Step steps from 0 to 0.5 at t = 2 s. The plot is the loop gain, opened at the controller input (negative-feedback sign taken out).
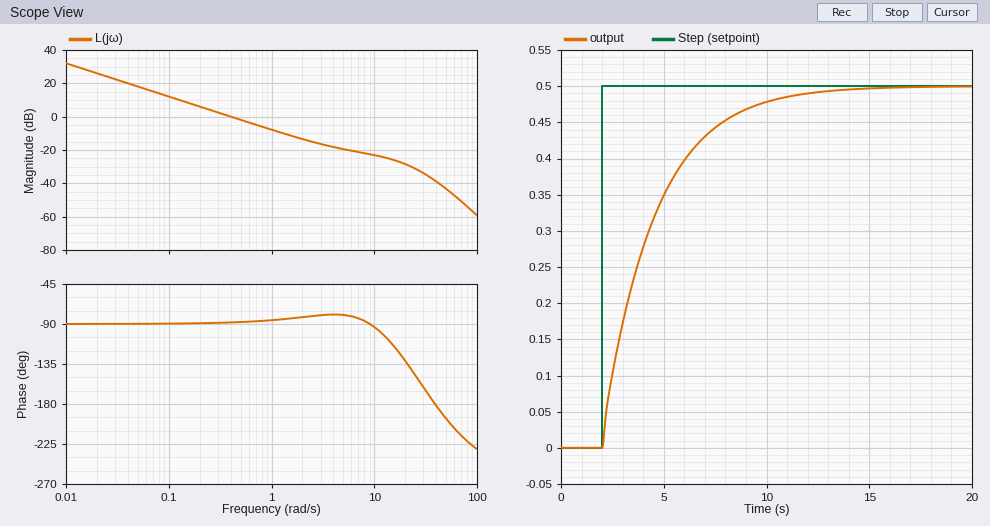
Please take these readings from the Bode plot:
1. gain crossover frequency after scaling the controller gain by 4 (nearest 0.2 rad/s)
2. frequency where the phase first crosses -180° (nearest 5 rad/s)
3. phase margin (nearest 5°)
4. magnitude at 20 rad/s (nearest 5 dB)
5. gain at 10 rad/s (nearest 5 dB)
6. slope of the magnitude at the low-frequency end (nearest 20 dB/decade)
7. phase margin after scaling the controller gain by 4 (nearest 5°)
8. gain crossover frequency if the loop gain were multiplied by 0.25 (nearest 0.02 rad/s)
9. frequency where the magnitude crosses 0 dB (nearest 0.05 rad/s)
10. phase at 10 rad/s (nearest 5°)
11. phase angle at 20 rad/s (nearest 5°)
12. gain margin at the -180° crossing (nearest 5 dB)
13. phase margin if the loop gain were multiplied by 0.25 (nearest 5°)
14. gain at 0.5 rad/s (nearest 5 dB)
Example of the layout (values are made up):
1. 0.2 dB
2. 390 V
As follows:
1. 1.6 rad/s
2. 40 rad/s
3. 90°
4. -30 dB
5. -25 dB
6. -20 dB/decade
7. 95°
8. 0.10 rad/s
9. 0.40 rad/s
10. -95°
11. -130°
12. 40 dB
13. 90°
14. 0 dB
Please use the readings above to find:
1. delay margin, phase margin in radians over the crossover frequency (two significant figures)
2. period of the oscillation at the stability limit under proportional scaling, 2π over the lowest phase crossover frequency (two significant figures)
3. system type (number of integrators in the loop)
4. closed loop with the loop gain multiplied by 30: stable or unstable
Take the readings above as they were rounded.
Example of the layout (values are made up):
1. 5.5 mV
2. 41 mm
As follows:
1. 3.9 s
2. 0.16 s
3. 1
4. stable
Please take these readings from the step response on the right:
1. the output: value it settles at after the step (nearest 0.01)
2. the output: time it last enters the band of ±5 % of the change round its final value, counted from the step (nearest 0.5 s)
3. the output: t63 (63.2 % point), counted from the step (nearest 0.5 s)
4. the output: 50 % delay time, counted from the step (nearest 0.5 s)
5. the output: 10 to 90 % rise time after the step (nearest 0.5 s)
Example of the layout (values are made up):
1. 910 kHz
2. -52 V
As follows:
1. 0.50
2. 7.5 s
3. 2.5 s
4. 1.5 s
5. 5.5 s
